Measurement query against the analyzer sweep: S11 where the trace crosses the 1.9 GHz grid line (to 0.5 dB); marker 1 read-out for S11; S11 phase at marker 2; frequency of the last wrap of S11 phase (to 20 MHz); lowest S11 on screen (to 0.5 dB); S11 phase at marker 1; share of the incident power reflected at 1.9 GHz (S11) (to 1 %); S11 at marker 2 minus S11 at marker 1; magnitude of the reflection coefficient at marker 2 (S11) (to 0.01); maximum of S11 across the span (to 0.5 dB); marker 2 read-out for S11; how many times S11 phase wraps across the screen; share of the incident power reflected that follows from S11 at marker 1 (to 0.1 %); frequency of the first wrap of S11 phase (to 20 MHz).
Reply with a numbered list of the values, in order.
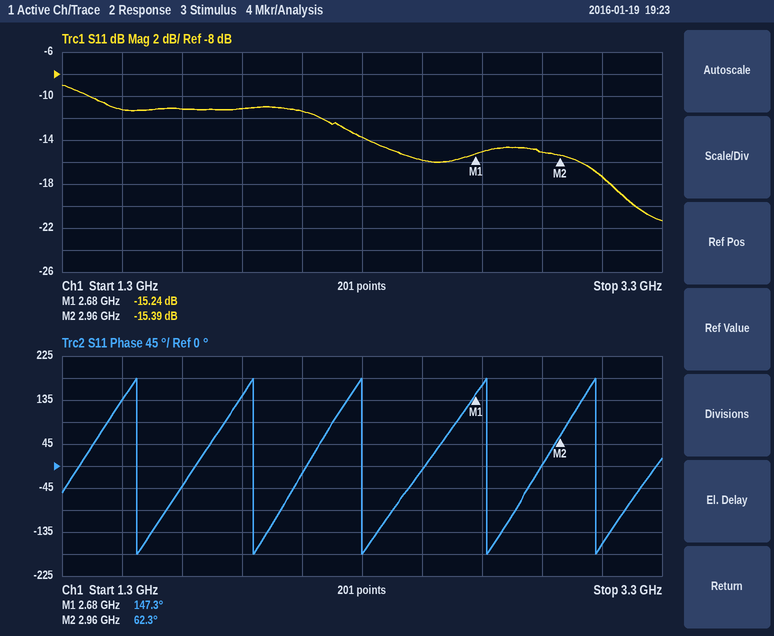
1. -11.0 dB
2. -15.24 dB
3. 62.3°
4. 3.08 GHz
5. -21.5 dB
6. 147.3°
7. 8 %
8. -0.15 dB
9. 0.17
10. -9.0 dB
11. -15.39 dB
12. 5
13. 3.0 %
14. 1.54 GHz
